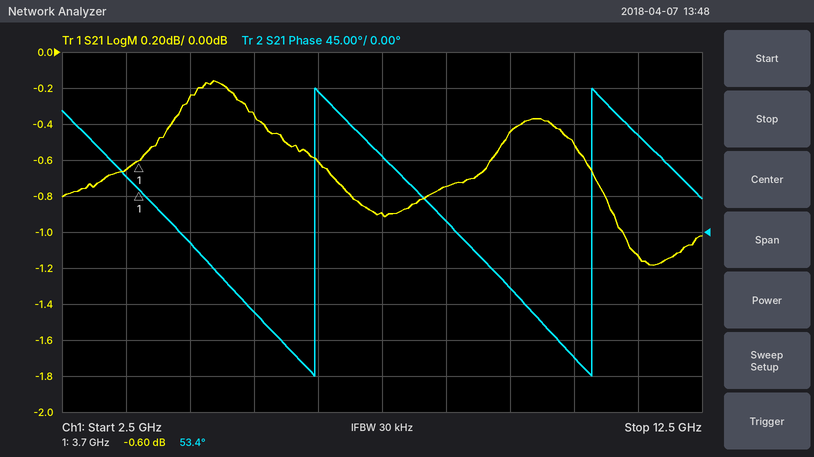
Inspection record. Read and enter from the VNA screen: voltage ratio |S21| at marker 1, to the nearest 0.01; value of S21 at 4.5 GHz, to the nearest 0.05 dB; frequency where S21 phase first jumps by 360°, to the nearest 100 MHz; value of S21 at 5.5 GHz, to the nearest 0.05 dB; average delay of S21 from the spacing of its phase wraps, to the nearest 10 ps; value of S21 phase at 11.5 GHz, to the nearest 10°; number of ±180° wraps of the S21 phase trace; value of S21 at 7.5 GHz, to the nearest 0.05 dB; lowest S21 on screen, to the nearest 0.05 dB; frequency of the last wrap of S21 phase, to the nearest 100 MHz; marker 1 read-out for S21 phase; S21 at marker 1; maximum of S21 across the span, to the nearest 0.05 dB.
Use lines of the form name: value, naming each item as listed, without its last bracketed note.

voltage ratio |S21| at marker 1, to the nearest 0.01: 0.93
value of S21 at 4.5 GHz, to the nearest 0.05 dB: -0.25 dB
frequency where S21 phase first jumps by 360°, to the nearest 100 MHz: 6.4 GHz
value of S21 at 5.5 GHz, to the nearest 0.05 dB: -0.35 dB
average delay of S21 from the spacing of its phase wraps, to the nearest 10 ps: 230 ps
value of S21 phase at 11.5 GHz, to the nearest 10°: 120°
number of ±180° wraps of the S21 phase trace: 2
value of S21 at 7.5 GHz, to the nearest 0.05 dB: -0.90 dB
lowest S21 on screen, to the nearest 0.05 dB: -1.20 dB
frequency of the last wrap of S21 phase, to the nearest 100 MHz: 10.8 GHz
marker 1 read-out for S21 phase: 53.4°
S21 at marker 1: -0.60 dB
maximum of S21 across the span, to the nearest 0.05 dB: -0.15 dB
